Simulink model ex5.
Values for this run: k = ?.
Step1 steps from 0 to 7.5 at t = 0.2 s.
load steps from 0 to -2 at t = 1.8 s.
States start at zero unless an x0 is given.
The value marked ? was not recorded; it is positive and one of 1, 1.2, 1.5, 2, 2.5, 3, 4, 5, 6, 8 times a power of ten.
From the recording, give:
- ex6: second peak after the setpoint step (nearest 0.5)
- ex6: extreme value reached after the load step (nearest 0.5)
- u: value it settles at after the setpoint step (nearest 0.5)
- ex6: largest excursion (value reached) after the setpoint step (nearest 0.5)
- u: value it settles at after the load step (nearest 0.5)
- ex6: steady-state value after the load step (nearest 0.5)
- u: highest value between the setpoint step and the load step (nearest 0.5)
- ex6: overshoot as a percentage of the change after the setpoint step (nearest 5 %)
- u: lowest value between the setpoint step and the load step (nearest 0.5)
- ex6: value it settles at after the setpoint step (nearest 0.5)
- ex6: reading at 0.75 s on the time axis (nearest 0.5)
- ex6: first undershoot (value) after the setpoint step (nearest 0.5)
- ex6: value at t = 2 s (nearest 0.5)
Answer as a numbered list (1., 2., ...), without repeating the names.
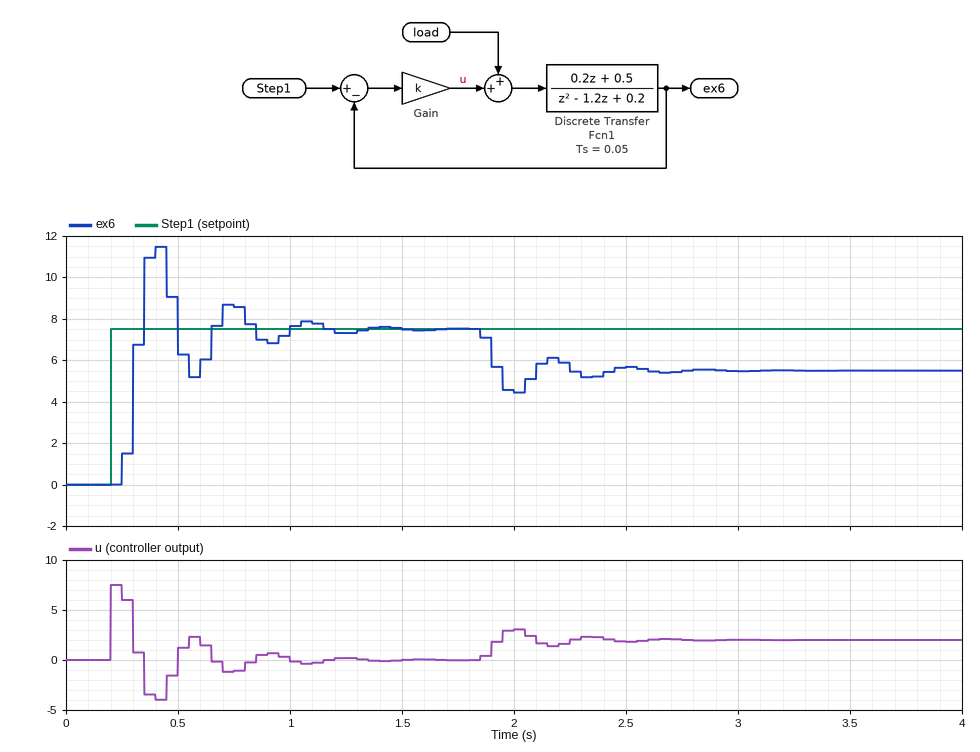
1. 8.5
2. 4.5
3. 0.0
4. 11.5
5. 2.0
6. 5.5
7. 7.5
8. 55 %
9. -4.0
10. 7.5
11. 8.5
12. 5.0
13. 4.5
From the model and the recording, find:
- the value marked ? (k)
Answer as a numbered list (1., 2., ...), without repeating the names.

1. 1
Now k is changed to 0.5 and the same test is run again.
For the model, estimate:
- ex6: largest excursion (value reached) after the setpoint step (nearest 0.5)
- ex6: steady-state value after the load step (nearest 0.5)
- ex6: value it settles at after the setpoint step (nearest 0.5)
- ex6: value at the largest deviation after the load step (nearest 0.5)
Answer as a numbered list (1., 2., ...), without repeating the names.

1. 8.5
2. 3.5
3. 7.5
4. 3.0
